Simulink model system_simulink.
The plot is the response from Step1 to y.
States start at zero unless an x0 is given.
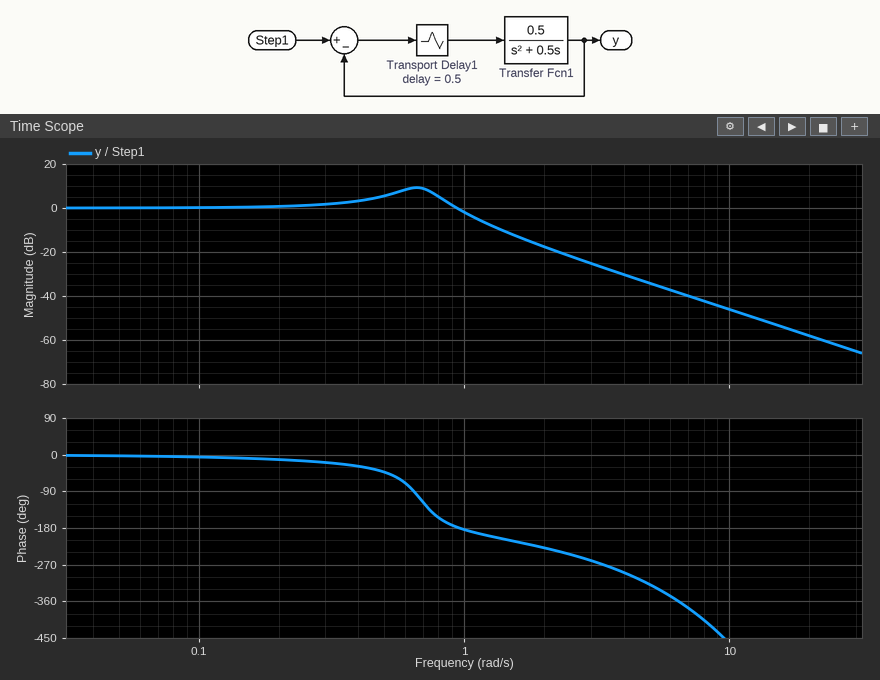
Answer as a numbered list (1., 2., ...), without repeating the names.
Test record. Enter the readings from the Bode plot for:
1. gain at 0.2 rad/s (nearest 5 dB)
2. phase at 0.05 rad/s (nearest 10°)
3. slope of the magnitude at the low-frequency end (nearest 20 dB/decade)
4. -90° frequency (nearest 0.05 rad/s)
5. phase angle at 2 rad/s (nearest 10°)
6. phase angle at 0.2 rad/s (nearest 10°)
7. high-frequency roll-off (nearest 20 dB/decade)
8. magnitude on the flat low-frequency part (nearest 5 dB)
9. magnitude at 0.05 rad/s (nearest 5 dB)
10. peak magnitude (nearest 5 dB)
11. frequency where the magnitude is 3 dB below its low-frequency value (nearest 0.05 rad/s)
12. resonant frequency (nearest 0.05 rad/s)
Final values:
1. 0 dB
2. 0°
3. 0 dB/decade
4. 0.65 rad/s
5. -230°
6. -10°
7. -40 dB/decade
8. 0 dB
9. 0 dB
10. 10 dB
11. 1.05 rad/s
12. 0.65 rad/s
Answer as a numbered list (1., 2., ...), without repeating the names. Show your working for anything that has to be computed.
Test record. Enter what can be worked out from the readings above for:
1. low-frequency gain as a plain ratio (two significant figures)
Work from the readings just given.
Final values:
1. 10^(0 / 20) = 1.0
